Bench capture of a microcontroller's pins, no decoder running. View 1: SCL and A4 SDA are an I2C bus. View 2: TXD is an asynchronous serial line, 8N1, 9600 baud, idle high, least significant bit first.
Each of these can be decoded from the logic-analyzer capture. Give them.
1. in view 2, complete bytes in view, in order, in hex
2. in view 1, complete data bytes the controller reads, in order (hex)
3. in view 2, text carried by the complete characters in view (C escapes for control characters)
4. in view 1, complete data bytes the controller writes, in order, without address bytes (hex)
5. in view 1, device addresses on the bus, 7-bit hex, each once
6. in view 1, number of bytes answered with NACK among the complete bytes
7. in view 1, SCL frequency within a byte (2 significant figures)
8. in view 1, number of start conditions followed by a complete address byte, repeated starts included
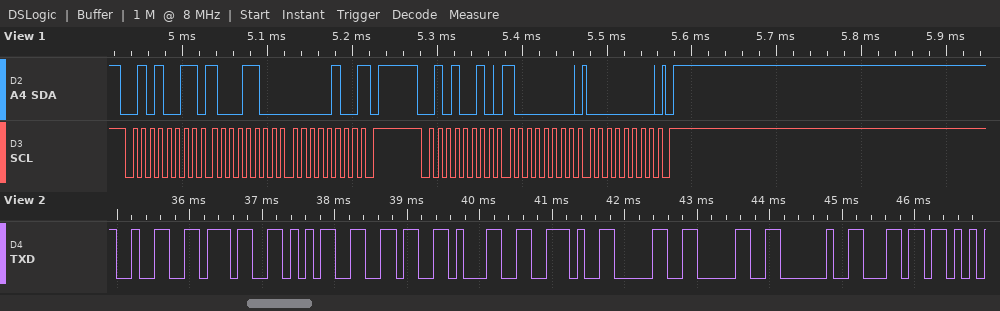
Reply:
32 37 35 36 31 2E 30 30 20 6C
8C 04
"27561.00 l"
80 00
0x29
1
100 kHz
2
